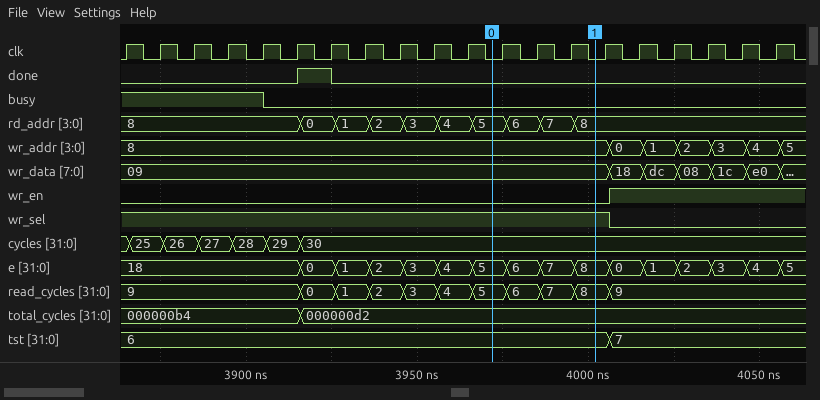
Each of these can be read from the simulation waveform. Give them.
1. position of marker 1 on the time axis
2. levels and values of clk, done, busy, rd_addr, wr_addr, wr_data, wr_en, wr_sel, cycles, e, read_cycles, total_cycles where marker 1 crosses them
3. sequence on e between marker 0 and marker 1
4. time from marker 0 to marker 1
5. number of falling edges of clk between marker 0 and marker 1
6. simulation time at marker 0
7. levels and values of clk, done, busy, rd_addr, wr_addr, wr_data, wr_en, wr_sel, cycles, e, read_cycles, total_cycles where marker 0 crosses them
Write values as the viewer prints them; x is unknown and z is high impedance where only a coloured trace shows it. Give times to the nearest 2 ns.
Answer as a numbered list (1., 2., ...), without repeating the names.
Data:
1. 4002 ns
2. clk=0, done=0, busy=0, rd_addr=8, wr_addr=8, wr_data=09, wr_en=0, wr_sel=1, cycles=30, e=8, read_cycles=8, total_cycles=000000d2
3. 5, 6, 7, 8
4. 30 ns
5. 3
6. 3972 ns
7. clk=0, done=0, busy=0, rd_addr=5, wr_addr=8, wr_data=09, wr_en=0, wr_sel=1, cycles=30, e=5, read_cycles=5, total_cycles=000000d2
